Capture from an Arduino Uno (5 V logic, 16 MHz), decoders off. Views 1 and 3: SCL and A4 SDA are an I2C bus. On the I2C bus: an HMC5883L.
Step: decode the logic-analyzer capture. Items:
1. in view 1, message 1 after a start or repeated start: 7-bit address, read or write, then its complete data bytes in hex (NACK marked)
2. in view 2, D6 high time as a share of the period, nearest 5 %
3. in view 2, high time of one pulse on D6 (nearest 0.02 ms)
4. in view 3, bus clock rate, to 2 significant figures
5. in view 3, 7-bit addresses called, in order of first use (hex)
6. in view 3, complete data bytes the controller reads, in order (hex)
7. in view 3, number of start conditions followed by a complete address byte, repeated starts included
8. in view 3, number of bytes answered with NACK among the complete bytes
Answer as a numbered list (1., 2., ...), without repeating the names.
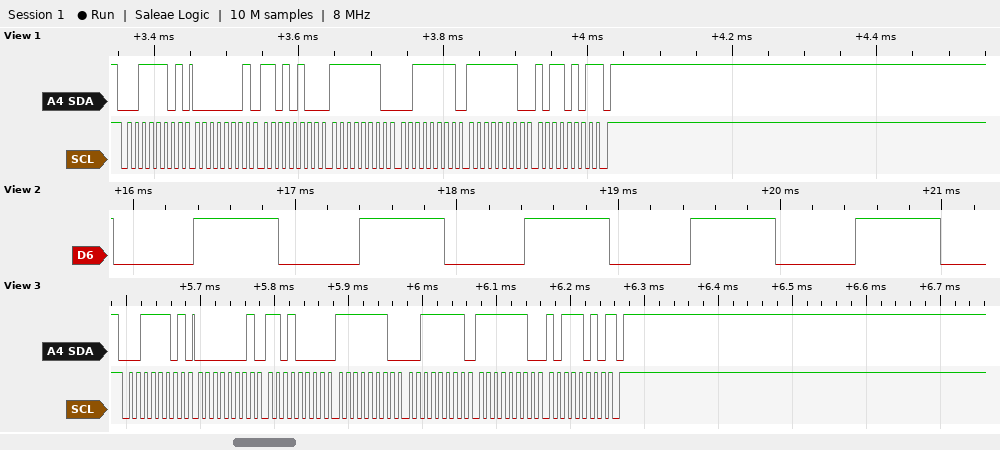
1. 0x1E read: 01 D4 FE 3F FE B5 NACK
2. 50 %
3. 0.52 ms
4. 100 kHz
5. 0x1E
6. 01 D0 FE 3F FE BA
7. 1
8. 1
